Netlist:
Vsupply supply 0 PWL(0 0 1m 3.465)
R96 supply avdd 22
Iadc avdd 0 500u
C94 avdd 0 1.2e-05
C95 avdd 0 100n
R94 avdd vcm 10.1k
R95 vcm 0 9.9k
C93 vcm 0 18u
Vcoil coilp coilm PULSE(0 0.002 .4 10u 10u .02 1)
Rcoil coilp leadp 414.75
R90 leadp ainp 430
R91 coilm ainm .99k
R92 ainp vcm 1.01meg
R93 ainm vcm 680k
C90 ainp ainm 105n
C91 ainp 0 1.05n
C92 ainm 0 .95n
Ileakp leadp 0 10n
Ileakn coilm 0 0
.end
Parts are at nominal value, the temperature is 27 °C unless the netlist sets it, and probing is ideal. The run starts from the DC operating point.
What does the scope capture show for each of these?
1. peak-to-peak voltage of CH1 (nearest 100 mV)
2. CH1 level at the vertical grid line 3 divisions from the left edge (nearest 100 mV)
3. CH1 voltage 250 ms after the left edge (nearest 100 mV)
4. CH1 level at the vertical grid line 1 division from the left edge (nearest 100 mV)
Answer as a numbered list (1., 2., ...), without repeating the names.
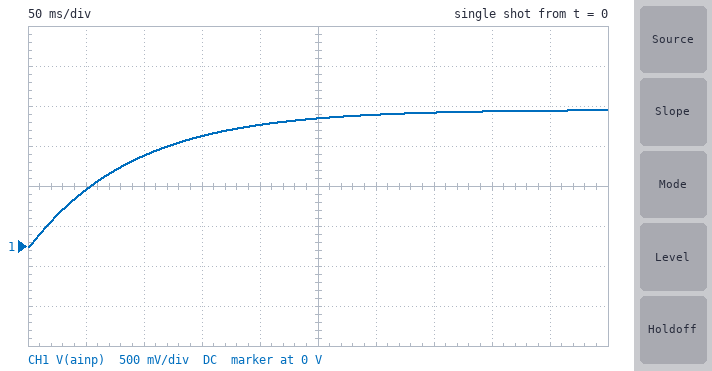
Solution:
1. 1.7 V
2. 1.4 V
3. 1.6 V
4. 700 mV
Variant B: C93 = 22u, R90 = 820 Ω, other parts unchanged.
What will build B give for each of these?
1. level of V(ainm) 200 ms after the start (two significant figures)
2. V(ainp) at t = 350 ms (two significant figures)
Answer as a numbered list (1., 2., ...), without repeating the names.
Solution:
1. 1.4 V
2. 1.6 V
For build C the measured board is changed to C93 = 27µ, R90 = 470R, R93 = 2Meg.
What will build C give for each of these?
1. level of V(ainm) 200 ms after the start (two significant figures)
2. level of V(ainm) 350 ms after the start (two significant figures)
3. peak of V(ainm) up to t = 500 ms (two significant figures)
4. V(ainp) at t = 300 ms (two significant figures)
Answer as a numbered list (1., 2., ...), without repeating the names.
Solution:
1. 1.3 V
2. 1.6 V
3. 1.7 V
4. 1.5 V
